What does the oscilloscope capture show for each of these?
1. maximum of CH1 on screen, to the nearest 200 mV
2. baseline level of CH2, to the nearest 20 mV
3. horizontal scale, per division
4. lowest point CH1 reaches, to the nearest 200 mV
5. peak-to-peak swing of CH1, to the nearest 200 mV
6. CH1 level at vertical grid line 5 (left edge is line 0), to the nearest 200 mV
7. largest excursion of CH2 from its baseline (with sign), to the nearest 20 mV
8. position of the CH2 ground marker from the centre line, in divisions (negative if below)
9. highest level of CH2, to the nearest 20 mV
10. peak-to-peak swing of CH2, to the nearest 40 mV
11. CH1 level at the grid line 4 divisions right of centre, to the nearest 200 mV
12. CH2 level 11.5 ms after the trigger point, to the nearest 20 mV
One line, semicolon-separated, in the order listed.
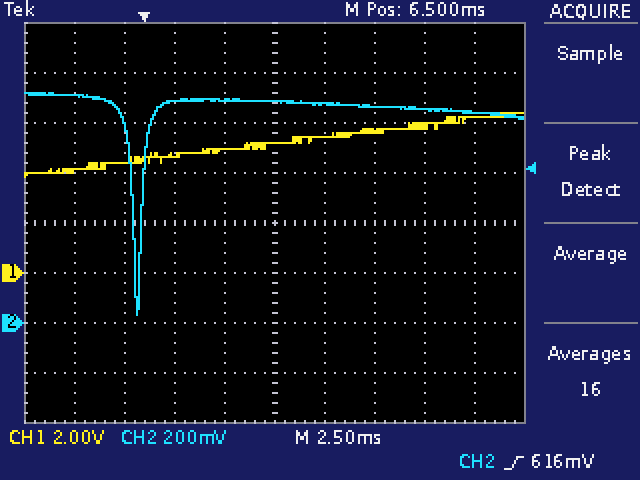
6.4 V; 880 mV; 2.5 ms; 3.8 V; 2.6 V; 5.2 V; -840 mV; -2.0 div; 920 mV; 880 mV; 6.2 V; 860 mV
